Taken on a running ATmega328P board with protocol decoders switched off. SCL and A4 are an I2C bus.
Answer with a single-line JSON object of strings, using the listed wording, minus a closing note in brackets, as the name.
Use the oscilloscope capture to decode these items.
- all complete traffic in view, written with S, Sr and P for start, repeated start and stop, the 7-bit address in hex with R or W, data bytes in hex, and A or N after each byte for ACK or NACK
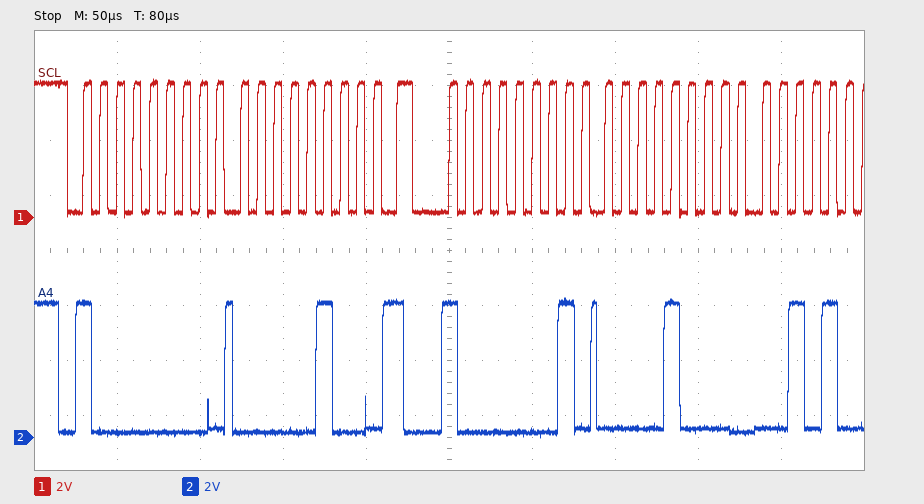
{"all complete traffic in view, written with S, Sr and P for start, repeated start and stop, the 7-bit address in hex with R or W, data bytes in hex, and A or N after each byte for ACK or NACK": "S 40W A 04 A Sr 40R A 08 A"}
